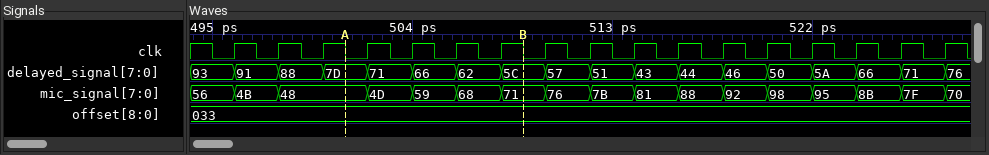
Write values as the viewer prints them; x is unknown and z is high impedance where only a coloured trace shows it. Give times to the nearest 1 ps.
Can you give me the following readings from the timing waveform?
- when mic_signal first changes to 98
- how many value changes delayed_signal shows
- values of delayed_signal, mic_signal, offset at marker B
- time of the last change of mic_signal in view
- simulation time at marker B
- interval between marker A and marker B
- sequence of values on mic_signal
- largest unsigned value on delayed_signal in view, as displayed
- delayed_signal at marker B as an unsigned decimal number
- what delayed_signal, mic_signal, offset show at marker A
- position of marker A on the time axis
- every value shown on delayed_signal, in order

520 ps
17
delayed_signal=5C, mic_signal=71, offset=033
528 ps
509 ps
8 ps
56, 4B, 48, 4D, 59, 68, 71, 76, 7B, 81, 88, 92, 98, 95, 8B, 7F, 70
93
92
delayed_signal=7D, mic_signal=48, offset=033
501 ps
93, 91, 88, 7D, 71, 66, 62, 5C, 57, 51, 43, 44, 46, 50, 5A, 66, 71, 76
